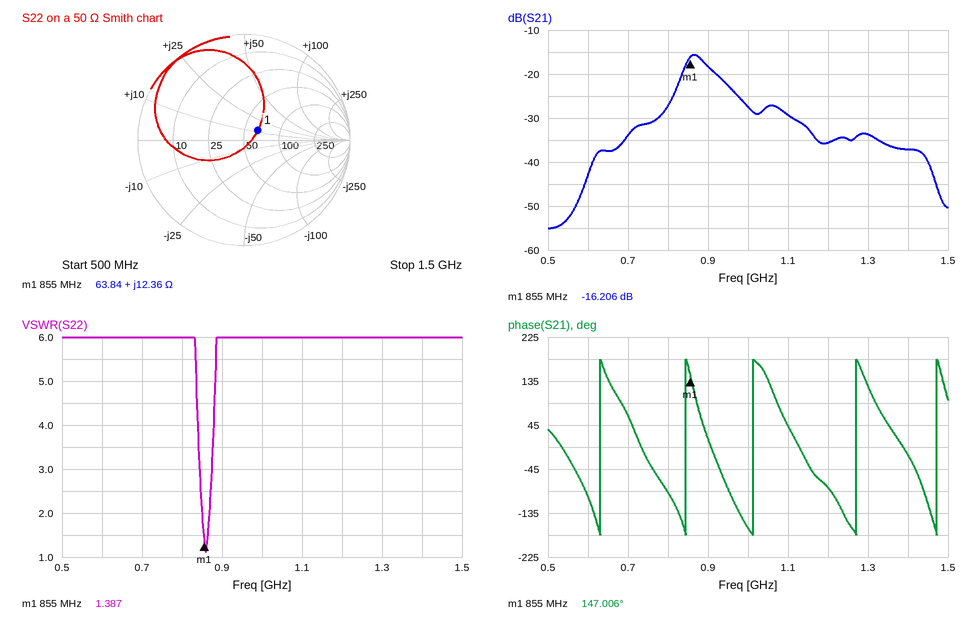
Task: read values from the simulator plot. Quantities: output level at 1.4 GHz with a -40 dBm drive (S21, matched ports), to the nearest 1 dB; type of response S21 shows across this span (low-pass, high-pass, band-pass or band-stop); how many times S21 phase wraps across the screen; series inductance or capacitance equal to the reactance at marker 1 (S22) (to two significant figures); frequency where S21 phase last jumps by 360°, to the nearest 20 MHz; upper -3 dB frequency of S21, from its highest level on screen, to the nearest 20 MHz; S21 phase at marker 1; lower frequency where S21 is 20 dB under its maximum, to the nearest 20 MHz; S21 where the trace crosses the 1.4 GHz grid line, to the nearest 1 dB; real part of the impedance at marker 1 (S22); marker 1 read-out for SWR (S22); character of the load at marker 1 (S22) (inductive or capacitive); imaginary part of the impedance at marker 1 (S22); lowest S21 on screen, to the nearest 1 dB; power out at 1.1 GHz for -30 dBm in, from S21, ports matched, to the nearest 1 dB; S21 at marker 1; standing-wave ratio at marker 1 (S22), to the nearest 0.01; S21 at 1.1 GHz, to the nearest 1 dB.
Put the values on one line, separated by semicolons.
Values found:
-77 dBm; band-pass; 5; 2.3 nH; 1.48 GHz; 900 MHz; 147.006°; 680 MHz; -37 dB; 63.84 Ω; 1.387; inductive; +12.36 Ω; -55 dB; -59 dBm; -16.206 dB; 1.39; -29 dB
